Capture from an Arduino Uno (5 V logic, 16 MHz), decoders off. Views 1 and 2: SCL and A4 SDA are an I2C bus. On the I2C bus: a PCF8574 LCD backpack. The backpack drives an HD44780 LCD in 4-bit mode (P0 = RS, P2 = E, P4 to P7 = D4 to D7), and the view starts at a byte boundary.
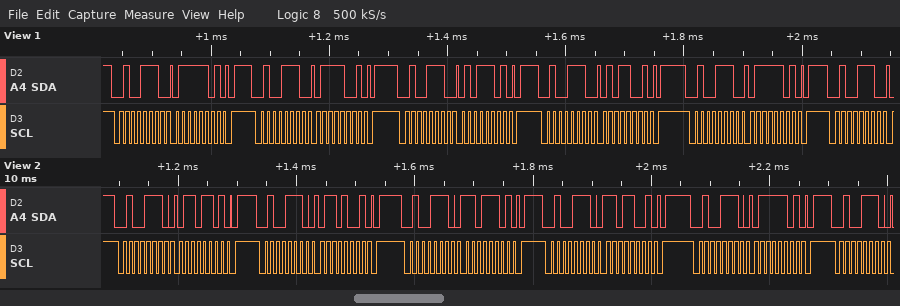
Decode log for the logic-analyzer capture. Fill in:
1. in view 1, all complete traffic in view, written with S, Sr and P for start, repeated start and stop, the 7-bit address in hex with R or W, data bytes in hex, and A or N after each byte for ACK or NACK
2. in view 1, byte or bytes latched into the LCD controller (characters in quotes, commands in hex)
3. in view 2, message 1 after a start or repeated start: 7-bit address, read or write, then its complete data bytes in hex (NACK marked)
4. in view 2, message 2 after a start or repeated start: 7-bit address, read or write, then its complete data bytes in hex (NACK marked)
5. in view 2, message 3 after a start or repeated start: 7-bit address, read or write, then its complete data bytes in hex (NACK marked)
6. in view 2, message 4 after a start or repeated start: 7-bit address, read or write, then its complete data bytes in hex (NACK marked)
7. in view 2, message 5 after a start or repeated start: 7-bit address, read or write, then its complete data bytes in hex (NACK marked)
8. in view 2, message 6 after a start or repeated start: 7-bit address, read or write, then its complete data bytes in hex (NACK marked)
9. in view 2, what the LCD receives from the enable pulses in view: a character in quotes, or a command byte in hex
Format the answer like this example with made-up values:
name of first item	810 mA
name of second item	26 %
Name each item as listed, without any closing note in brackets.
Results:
in view 1, all complete traffic in view, written with S, Sr and P for start, repeated start and stop, the 7-bit address in hex with R or W, data bytes in hex, and A or N after each byte for ACK or NACK	S 27W A 7D A P S 27W A 79 A P S 27W A 5D A P S 27W A 59 A P S 27W A 7D A P S 27W A
in view 1, byte or bytes latched into the LCD controller	'u'
in view 2, message 1 after a start or repeated start: 7-bit address, read or write, then its complete data bytes in hex	0x27 write: 6D
in view 2, message 2 after a start or repeated start: 7-bit address, read or write, then its complete data bytes in hex	0x27 write: 69
in view 2, message 3 after a start or repeated start: 7-bit address, read or write, then its complete data bytes in hex	0x27 write: DD
in view 2, message 4 after a start or repeated start: 7-bit address, read or write, then its complete data bytes in hex	0x27 write: D9
in view 2, message 5 after a start or repeated start: 7-bit address, read or write, then its complete data bytes in hex	0x27 write: 7D
in view 2, message 6 after a start or repeated start: 7-bit address, read or write, then its complete data bytes in hex	0x27 write
in view 2, what the LCD receives from the enable pulses in view: a character in quotes, or a command byte in hex	'm'
